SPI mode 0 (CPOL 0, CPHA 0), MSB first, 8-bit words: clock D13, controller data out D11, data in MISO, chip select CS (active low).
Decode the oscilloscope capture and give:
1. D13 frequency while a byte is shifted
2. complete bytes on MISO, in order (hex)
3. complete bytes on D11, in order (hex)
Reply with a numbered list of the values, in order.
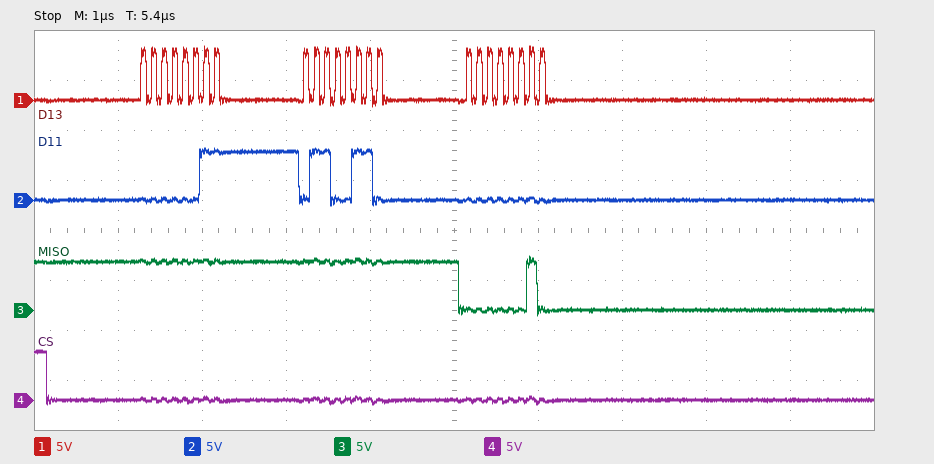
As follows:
1. 8 MHz
2. FF FF 02
3. 03 66 00
